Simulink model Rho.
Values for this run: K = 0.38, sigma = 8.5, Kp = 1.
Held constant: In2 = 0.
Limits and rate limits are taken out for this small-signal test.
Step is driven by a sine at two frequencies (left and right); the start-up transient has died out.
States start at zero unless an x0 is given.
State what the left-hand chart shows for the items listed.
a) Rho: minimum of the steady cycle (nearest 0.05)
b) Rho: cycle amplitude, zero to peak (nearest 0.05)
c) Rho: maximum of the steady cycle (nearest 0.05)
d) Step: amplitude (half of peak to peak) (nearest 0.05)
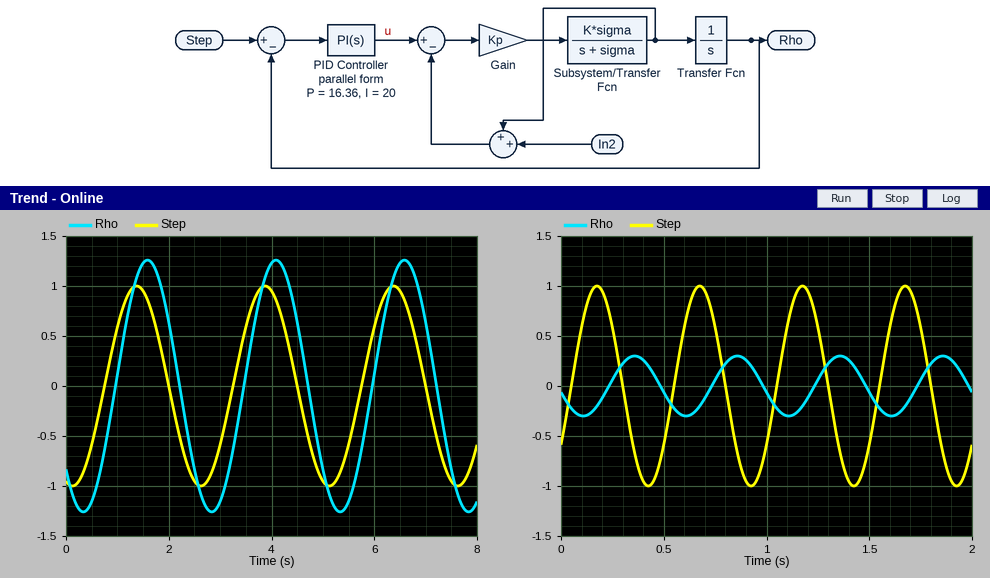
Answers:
-1.25
1.25
1.25
1.00
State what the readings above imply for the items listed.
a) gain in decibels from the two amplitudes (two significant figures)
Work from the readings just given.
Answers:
1.9 dB
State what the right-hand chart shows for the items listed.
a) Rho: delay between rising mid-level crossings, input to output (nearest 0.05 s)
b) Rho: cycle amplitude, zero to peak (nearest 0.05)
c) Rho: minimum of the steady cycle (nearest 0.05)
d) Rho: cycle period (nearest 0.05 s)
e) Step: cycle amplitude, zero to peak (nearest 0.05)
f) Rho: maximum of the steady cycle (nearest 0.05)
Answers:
0.20 s
0.30
-0.30
0.50 s
1.00
0.30
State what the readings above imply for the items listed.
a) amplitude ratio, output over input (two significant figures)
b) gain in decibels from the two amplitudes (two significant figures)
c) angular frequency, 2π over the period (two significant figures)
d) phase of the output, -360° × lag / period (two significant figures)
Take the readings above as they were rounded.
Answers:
0.30
-10 dB
13 rad/s
-140°
